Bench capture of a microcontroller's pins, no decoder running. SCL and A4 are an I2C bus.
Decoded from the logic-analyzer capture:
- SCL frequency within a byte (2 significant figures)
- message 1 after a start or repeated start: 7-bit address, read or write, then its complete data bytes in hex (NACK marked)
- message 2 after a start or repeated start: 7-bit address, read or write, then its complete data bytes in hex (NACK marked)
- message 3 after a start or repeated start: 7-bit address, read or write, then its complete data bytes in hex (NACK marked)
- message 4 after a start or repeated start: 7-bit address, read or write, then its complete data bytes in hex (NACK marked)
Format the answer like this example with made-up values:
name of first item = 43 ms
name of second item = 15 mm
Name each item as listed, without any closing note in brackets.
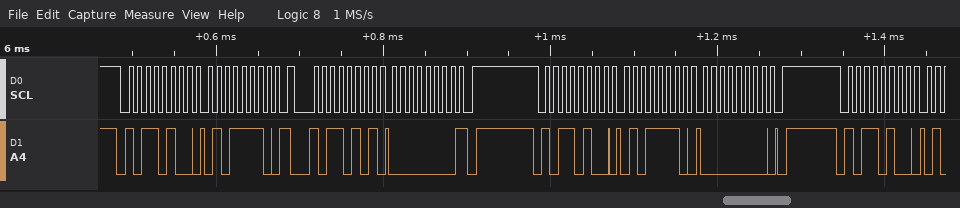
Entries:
SCL frequency within a byte = 100 kHz
message 1 after a start or repeated start: 7-bit address, read or write, then its complete data bytes in hex = 0x5A write: 5E
message 2 after a start or repeated start: 7-bit address, read or write, then its complete data bytes in hex = 0x5A read: 00 NACK
message 3 after a start or repeated start: 7-bit address, read or write, then its complete data bytes in hex = 0x5A write: 5E 00
message 4 after a start or repeated start: 7-bit address, read or write, then its complete data bytes in hex = 0x5A write
